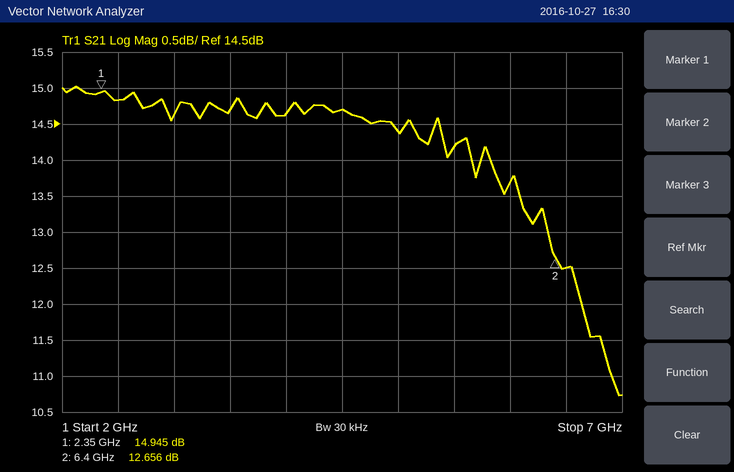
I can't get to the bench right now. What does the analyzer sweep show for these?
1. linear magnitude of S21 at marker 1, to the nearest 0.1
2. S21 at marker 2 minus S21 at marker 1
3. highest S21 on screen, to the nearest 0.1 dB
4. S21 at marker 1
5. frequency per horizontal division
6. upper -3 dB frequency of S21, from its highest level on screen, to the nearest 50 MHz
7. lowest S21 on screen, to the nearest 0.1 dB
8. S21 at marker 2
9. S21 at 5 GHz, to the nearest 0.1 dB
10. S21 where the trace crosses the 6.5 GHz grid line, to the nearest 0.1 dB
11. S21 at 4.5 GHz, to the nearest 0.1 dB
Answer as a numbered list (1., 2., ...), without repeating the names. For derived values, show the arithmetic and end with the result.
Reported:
1. 10^(14.945/20) ≈ 5.6
2. 12.656 − (14.945) = -2.289 dB
3. 15.0 dB
4. 14.945 dB
5. 500 MHz
6. 6.65 GHz
7. 10.7 dB
8. 12.656 dB
9. 14.4 dB
10. 12.5 dB
11. 14.7 dB
